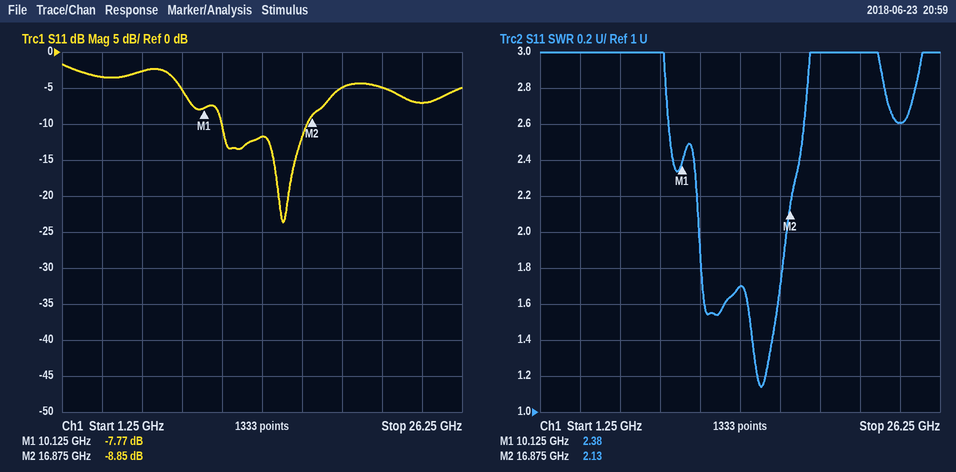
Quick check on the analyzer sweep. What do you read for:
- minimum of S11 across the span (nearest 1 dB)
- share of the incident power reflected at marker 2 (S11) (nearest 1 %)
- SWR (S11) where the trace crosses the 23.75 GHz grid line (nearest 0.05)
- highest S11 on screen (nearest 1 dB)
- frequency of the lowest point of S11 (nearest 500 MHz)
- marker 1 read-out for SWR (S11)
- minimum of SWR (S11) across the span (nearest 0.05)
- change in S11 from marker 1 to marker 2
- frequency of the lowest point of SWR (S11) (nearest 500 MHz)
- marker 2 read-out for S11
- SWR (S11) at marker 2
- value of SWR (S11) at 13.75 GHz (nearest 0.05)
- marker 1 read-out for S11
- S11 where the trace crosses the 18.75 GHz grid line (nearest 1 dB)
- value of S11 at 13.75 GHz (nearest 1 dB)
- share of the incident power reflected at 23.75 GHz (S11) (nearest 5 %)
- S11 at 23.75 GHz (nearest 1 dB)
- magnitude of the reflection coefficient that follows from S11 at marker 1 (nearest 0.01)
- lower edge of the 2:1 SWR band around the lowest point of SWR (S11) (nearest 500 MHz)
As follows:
-24 dB
13 %
2.60
-2 dB
15.0 GHz
2.38
1.15
-1.08 dB
15.0 GHz
-8.85 dB
2.13
1.70
-7.77 dB
-5 dB
-12 dB
20 %
-7 dB
0.41
11.0 GHz
